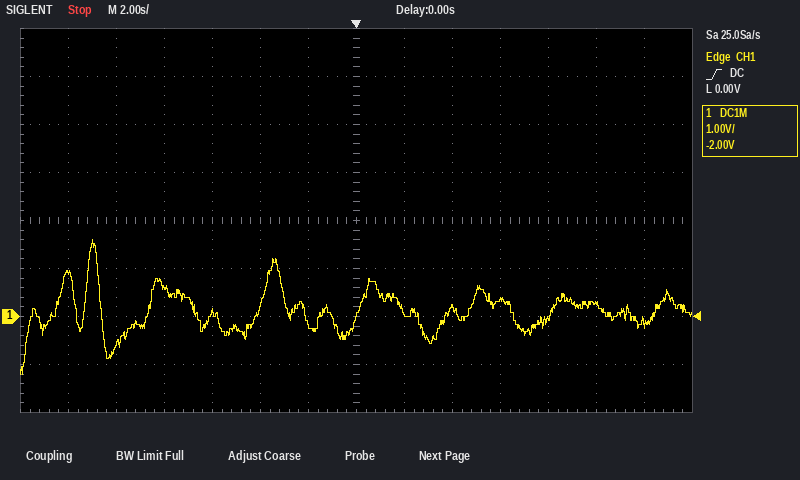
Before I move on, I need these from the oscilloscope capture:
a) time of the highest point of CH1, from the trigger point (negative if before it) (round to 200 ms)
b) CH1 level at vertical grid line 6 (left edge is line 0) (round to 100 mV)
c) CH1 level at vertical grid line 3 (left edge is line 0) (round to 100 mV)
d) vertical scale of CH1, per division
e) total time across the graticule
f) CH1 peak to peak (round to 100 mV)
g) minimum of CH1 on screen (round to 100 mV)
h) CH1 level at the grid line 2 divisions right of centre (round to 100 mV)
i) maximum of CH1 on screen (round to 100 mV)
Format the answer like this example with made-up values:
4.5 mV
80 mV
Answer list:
-11.0 s
-200 mV
600 mV
1 V
28 s
2.8 V
-1.2 V
200 mV
1.6 V
